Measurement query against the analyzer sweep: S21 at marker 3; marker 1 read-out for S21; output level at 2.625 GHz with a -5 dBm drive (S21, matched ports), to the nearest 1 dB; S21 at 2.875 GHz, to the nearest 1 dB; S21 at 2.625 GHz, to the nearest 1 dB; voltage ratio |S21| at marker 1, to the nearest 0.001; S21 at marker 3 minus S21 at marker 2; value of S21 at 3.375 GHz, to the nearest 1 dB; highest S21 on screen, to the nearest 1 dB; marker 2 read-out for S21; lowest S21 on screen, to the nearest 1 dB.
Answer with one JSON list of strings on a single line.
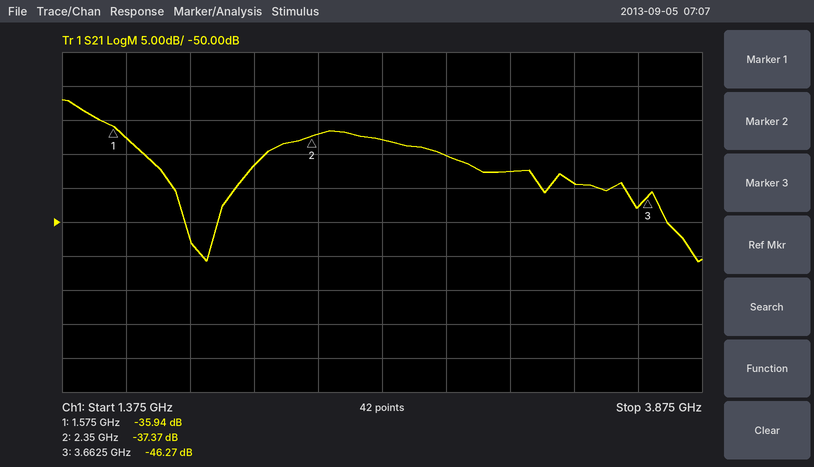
["-46.27 dB", "-35.94 dB", "-43 dBm", "-40 dB", "-38 dB", "0.016", "-8.90 dB", "-44 dB", "-32 dB", "-37.37 dB", "-56 dB"]
